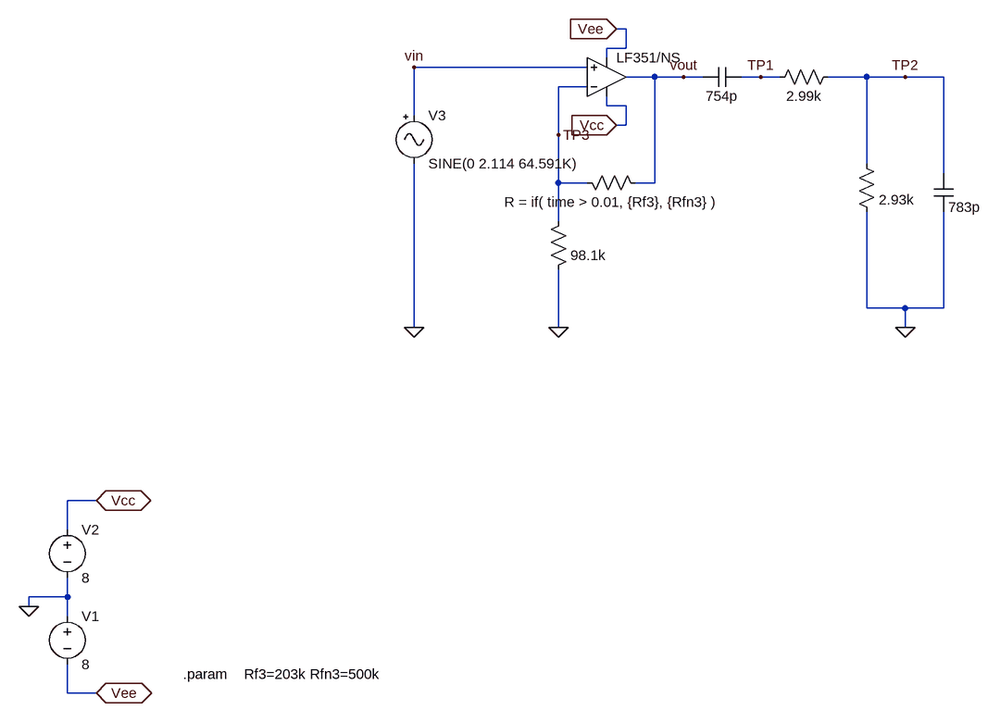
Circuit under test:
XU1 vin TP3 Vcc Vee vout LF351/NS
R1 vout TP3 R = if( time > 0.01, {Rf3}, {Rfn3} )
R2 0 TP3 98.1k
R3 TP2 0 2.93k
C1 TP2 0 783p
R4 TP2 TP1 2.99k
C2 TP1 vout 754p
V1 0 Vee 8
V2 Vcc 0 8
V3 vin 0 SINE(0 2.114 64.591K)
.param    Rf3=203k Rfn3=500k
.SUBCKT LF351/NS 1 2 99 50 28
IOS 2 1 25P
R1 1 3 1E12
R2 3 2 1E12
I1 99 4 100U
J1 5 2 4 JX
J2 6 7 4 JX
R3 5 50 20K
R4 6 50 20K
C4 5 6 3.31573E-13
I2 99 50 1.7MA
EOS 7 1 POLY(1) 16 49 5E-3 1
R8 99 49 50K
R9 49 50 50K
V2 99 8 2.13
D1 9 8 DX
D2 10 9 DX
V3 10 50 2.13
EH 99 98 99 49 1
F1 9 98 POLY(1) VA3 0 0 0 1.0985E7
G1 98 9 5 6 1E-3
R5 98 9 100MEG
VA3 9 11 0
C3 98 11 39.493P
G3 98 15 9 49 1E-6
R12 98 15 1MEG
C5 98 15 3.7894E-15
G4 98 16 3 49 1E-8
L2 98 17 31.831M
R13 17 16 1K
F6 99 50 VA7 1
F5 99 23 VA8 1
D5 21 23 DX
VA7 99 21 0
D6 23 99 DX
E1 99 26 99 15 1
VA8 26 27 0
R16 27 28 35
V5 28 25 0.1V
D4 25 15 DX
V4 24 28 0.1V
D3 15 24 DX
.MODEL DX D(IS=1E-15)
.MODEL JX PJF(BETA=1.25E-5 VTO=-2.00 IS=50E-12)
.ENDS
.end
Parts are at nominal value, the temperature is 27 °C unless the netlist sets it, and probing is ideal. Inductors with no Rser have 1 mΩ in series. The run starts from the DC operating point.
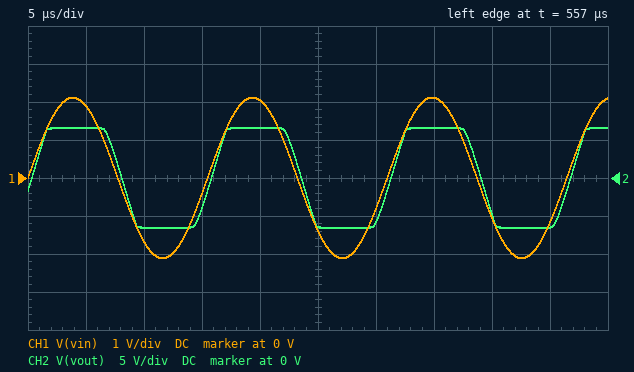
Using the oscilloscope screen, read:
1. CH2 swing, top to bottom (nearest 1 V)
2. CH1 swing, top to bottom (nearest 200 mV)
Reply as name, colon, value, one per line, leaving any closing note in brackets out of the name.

CH2 swing, top to bottom: 13 V
CH1 swing, top to bottom: 4.2 V
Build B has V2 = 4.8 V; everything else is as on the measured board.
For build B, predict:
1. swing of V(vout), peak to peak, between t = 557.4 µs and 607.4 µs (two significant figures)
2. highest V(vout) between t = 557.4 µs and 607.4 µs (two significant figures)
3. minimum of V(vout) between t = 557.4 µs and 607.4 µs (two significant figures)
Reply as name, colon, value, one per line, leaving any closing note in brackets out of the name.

swing of V(vout), peak to peak, between t = 557.4 µs and 607.4 µs: 9.9 V
highest V(vout) between t = 557.4 µs and 607.4 µs: 3.4 V
minimum of V(vout) between t = 557.4 µs and 607.4 µs: -6.6 V
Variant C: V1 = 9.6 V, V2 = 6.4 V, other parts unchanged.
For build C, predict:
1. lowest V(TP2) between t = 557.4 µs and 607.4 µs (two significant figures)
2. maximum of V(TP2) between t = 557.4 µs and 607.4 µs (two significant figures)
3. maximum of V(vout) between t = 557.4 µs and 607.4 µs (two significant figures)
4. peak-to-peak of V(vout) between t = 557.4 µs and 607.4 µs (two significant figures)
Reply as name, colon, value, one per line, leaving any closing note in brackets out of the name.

lowest V(TP2) between t = 557.4 µs and 607.4 µs: -2.6 V
maximum of V(TP2) between t = 557.4 µs and 607.4 µs: 2.4 V
maximum of V(vout) between t = 557.4 µs and 607.4 µs: 5.0 V
peak-to-peak of V(vout) between t = 557.4 µs and 607.4 µs: 13 V
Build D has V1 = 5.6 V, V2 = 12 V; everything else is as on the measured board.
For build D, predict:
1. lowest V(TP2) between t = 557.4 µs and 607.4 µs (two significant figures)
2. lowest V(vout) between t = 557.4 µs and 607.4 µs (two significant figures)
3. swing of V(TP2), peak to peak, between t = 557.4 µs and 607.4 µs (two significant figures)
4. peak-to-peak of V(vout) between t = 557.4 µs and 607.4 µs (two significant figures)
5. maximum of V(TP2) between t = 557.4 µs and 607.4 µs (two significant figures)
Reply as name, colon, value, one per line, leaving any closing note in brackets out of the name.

lowest V(TP2) between t = 557.4 µs and 607.4 µs: -2.5 V
lowest V(vout) between t = 557.4 µs and 607.4 µs: -4.2 V
swing of V(TP2), peak to peak, between t = 557.4 µs and 607.4 µs: 5.5 V
peak-to-peak of V(vout) between t = 557.4 µs and 607.4 µs: 15 V
maximum of V(TP2) between t = 557.4 µs and 607.4 µs: 3.0 V
